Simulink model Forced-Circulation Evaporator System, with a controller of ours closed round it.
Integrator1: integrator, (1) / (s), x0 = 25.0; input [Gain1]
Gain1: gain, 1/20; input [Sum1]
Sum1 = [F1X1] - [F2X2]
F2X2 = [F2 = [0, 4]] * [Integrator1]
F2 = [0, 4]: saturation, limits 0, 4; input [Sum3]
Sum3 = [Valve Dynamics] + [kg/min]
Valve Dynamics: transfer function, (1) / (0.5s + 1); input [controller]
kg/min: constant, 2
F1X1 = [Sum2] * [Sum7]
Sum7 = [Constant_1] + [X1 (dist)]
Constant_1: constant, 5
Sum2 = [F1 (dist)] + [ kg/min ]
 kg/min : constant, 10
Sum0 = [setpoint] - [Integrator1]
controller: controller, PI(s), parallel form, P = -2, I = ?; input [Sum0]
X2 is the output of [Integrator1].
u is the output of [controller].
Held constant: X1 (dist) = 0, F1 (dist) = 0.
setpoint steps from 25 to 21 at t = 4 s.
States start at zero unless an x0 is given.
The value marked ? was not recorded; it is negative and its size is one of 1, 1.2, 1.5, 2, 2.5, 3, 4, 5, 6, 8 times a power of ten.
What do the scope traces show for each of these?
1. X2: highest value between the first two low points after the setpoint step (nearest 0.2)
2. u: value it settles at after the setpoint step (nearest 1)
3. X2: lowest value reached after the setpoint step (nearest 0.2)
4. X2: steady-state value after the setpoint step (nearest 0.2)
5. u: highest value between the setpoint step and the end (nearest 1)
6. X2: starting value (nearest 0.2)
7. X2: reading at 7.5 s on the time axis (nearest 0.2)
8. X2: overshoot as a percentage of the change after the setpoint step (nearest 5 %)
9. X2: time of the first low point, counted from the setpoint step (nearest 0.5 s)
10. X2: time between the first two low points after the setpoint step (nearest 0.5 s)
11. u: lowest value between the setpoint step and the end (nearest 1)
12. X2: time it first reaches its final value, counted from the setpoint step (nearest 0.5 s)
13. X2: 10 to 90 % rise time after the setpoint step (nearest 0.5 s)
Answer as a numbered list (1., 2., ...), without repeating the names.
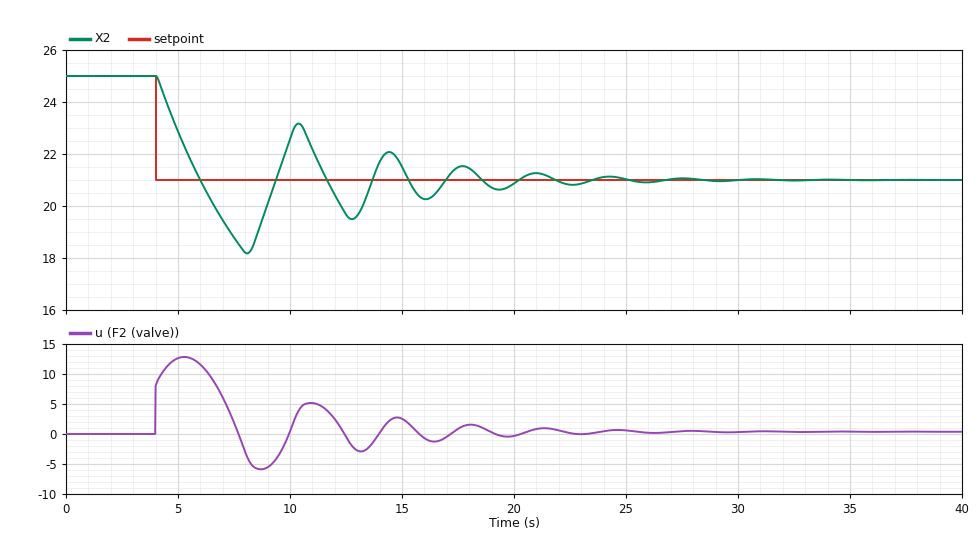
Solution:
1. 23.2
2. 0
3. 18.2
4. 21.0
5. 13
6. 25.0
7. 18.8
8. 70 %
9. 4.0 s
10. 4.5 s
11. -6
12. 2.0 s
13. 1.5 s
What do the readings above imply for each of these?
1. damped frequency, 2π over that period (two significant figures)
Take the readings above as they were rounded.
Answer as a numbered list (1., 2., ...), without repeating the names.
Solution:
1. 1.4 rad/s
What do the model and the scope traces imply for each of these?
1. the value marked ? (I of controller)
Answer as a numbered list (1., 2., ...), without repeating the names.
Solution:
1. -3
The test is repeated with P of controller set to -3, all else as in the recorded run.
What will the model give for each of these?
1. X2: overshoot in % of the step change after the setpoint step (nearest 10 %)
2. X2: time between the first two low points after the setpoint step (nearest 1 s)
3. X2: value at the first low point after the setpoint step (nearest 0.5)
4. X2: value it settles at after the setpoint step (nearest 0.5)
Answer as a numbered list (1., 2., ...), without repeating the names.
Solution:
1. 60 %
2. 3 s
3. 18.5
4. 21.0
